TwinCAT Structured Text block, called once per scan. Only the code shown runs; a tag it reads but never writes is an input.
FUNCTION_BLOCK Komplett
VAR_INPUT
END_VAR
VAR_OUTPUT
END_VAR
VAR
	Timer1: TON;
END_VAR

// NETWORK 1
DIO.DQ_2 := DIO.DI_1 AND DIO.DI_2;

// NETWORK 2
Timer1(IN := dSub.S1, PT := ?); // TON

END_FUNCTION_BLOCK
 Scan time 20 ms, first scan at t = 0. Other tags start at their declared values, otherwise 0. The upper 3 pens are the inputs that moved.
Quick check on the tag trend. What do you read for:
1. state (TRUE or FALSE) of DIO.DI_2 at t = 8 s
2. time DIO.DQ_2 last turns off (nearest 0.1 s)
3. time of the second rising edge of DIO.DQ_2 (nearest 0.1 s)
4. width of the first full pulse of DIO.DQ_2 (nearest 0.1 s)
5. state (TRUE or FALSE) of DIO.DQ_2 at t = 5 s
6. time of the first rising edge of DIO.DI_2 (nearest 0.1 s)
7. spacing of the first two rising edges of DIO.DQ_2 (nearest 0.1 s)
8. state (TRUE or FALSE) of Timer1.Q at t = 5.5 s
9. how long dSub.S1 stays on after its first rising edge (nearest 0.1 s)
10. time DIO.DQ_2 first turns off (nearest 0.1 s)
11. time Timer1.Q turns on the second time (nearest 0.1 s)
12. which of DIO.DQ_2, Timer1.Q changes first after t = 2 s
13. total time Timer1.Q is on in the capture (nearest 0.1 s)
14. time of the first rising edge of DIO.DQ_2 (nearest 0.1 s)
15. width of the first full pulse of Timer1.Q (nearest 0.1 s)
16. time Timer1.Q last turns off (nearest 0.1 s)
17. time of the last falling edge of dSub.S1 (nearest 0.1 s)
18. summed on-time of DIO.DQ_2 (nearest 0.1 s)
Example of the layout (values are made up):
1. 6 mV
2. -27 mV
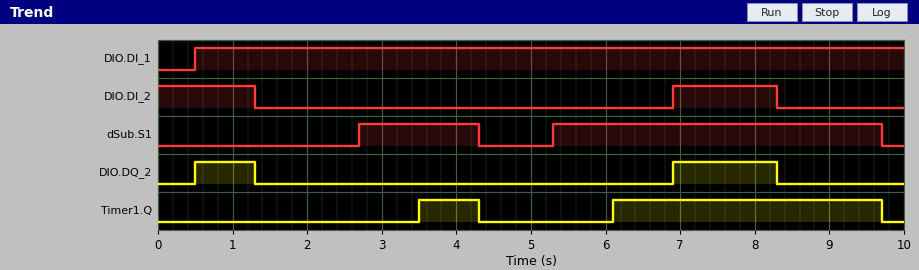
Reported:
1. TRUE
2. 8.3 s
3. 6.9 s
4. 0.8 s
5. FALSE
6. 6.9 s
7. 6.4 s
8. FALSE
9. 1.6 s
10. 1.3 s
11. 6.1 s
12. Timer1.Q
13. 4.4 s
14. 0.5 s
15. 0.8 s
16. 9.7 s
17. 9.7 s
18. 2.2 s
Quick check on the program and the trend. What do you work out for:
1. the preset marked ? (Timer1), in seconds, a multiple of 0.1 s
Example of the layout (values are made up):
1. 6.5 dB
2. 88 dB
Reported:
1. 0.8 s
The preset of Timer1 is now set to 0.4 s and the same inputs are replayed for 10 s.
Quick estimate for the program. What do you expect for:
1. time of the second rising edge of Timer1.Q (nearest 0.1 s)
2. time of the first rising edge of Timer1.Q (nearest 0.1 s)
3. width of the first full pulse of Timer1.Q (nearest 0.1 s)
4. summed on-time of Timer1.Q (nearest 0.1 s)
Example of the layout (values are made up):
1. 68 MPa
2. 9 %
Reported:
1. 5.7 s
2. 3.1 s
3. 1.2 s
4. 5.2 s
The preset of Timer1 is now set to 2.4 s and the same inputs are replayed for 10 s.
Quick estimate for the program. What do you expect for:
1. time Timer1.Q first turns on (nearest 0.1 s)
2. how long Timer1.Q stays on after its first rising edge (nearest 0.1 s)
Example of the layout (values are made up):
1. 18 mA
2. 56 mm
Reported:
1. 7.7 s
2. 2.0 s
